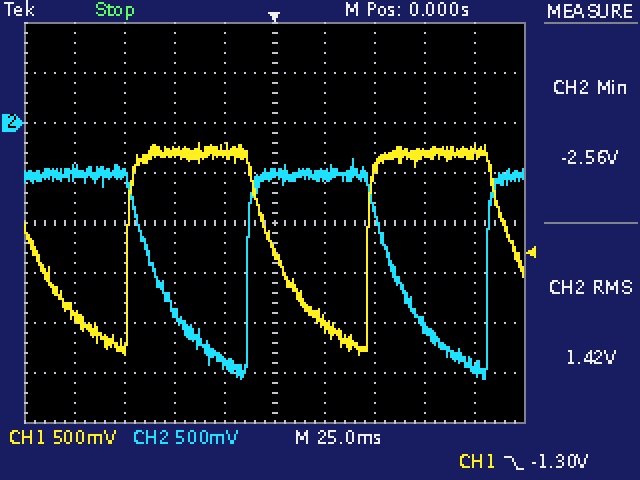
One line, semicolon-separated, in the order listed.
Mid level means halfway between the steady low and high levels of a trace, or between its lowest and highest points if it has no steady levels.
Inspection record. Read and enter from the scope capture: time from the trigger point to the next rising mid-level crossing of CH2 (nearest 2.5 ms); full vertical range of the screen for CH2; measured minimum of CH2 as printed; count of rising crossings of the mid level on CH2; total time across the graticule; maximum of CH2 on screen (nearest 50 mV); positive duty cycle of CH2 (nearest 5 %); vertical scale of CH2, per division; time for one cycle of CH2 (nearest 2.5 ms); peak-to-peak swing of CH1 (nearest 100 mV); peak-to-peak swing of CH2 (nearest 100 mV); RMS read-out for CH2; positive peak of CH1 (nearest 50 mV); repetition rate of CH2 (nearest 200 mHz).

107.5 ms; 4 V; -2.56 V; 2; 250 ms; -350 mV; 60 %; 500 mV; 120.0 ms; 2.10 V; 2.20 V; 1.42 V; -200 mV; 8.4 Hz
